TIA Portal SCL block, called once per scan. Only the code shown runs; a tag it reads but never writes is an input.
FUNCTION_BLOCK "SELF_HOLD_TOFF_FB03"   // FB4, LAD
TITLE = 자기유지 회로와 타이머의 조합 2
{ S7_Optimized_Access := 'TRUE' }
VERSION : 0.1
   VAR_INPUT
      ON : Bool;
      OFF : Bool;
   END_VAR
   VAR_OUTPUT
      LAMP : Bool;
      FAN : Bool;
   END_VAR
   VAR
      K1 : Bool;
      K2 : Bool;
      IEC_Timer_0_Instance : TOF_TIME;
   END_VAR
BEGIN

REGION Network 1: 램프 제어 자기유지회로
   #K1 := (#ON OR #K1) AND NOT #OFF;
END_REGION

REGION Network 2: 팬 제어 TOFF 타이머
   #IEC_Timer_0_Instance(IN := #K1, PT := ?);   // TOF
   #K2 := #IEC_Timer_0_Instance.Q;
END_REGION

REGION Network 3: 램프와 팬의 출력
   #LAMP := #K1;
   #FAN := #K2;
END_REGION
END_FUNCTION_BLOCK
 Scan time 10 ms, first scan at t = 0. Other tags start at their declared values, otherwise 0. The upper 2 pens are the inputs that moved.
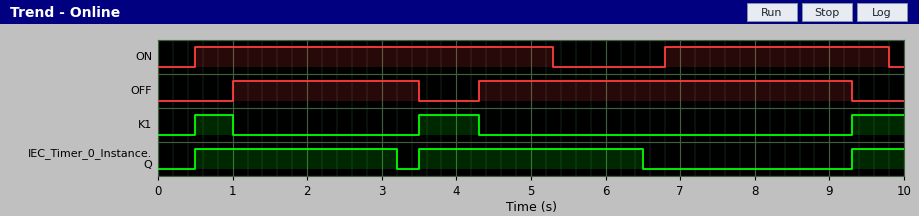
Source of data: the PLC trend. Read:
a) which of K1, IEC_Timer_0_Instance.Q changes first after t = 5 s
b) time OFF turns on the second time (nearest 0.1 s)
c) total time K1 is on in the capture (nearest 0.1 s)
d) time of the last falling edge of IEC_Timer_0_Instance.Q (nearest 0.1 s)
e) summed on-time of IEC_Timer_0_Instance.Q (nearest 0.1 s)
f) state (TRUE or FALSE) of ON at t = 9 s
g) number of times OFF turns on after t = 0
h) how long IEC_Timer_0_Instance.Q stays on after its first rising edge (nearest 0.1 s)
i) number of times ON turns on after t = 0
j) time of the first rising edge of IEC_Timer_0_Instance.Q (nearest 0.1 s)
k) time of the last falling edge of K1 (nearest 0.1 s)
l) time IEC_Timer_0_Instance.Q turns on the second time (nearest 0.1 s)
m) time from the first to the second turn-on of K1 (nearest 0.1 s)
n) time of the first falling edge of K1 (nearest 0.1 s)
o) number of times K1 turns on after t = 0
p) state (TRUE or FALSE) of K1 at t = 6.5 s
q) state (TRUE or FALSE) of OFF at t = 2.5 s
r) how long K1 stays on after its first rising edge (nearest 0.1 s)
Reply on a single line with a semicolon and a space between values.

IEC_Timer_0_Instance.Q; 4.3 s; 2.0 s; 6.5 s; 6.4 s; TRUE; 2; 2.7 s; 2; 0.5 s; 4.3 s; 3.5 s; 3.0 s; 1.0 s; 3; FALSE; TRUE; 0.5 s
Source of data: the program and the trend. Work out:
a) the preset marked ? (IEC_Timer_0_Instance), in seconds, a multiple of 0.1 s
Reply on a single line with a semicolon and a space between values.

2.2 s
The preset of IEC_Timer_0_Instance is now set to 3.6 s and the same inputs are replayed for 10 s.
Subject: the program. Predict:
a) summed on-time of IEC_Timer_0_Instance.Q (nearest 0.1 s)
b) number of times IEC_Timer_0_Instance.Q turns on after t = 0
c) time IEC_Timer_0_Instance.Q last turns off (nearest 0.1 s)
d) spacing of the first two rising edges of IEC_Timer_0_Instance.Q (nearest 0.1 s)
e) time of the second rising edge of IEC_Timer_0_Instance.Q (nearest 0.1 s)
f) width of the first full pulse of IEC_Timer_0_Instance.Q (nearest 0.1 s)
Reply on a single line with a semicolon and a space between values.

8.1 s; 2; 7.9 s; 8.8 s; 9.3 s; 7.4 s
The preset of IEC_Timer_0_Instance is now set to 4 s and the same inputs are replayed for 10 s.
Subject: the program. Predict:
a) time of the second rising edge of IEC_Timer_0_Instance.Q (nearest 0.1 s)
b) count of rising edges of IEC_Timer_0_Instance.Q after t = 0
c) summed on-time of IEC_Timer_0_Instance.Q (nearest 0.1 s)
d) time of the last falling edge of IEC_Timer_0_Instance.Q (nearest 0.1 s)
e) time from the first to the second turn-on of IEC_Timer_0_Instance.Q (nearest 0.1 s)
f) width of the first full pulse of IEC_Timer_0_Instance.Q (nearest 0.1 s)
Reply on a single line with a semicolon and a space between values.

9.3 s; 2; 8.5 s; 8.3 s; 8.8 s; 7.8 s
